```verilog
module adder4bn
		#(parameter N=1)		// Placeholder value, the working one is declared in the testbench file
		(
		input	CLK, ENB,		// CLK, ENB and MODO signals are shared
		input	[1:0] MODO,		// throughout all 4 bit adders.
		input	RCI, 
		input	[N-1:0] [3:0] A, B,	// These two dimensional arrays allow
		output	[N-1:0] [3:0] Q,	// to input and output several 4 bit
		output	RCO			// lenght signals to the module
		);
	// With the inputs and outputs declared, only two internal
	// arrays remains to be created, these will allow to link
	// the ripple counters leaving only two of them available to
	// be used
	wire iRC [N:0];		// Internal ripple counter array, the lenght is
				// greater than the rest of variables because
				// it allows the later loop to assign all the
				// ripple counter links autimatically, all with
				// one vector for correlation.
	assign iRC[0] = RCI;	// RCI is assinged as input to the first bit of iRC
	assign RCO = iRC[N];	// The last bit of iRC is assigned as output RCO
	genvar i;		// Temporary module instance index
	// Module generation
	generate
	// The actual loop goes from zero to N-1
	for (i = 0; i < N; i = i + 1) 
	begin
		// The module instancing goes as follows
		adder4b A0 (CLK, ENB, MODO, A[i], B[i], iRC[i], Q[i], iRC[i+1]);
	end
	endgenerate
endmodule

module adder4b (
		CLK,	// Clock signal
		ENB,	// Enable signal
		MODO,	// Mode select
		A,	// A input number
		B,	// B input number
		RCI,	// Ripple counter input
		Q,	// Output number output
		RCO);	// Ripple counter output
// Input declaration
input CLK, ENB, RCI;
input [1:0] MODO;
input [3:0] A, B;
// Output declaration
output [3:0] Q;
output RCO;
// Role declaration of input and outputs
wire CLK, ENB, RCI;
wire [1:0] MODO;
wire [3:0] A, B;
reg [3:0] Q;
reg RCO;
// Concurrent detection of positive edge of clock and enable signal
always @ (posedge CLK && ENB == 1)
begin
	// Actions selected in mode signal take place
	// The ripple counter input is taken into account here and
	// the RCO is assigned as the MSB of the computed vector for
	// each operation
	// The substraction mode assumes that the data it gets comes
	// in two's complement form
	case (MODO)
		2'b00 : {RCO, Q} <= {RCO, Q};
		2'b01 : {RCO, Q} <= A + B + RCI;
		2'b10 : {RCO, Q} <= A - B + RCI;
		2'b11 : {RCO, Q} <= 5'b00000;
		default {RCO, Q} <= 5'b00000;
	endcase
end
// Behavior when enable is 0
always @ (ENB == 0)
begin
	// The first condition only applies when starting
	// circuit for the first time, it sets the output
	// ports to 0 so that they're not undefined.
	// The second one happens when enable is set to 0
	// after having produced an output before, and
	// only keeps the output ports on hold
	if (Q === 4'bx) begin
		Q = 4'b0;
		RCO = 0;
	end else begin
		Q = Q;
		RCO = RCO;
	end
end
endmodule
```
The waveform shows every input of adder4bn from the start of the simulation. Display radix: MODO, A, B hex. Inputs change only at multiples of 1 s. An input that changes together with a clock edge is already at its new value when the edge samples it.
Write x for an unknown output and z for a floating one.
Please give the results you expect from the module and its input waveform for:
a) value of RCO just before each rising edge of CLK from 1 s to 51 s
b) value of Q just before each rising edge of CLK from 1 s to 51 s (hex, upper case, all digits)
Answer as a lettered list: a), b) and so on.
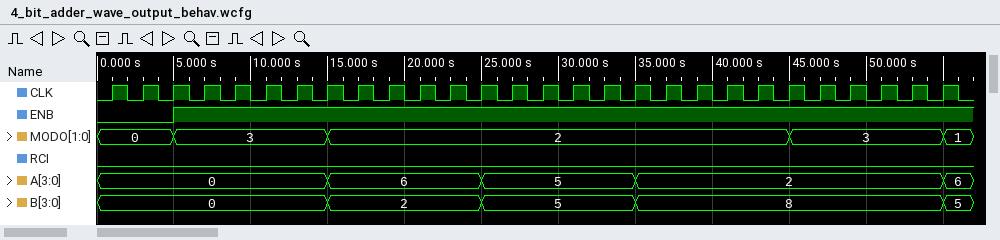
a) 0 0 0 0 0 0 0 0 0 0 0 0 0 0 0 0 0 0 1 1 1 1 1 0 0 0
b) 0, 0, 0, 0, 0, 0, 0, 0, 4, 4, 4, 4, 4, 0, 0, 0, 0, 0, A, A, A, A, A, 0, 0, 0
